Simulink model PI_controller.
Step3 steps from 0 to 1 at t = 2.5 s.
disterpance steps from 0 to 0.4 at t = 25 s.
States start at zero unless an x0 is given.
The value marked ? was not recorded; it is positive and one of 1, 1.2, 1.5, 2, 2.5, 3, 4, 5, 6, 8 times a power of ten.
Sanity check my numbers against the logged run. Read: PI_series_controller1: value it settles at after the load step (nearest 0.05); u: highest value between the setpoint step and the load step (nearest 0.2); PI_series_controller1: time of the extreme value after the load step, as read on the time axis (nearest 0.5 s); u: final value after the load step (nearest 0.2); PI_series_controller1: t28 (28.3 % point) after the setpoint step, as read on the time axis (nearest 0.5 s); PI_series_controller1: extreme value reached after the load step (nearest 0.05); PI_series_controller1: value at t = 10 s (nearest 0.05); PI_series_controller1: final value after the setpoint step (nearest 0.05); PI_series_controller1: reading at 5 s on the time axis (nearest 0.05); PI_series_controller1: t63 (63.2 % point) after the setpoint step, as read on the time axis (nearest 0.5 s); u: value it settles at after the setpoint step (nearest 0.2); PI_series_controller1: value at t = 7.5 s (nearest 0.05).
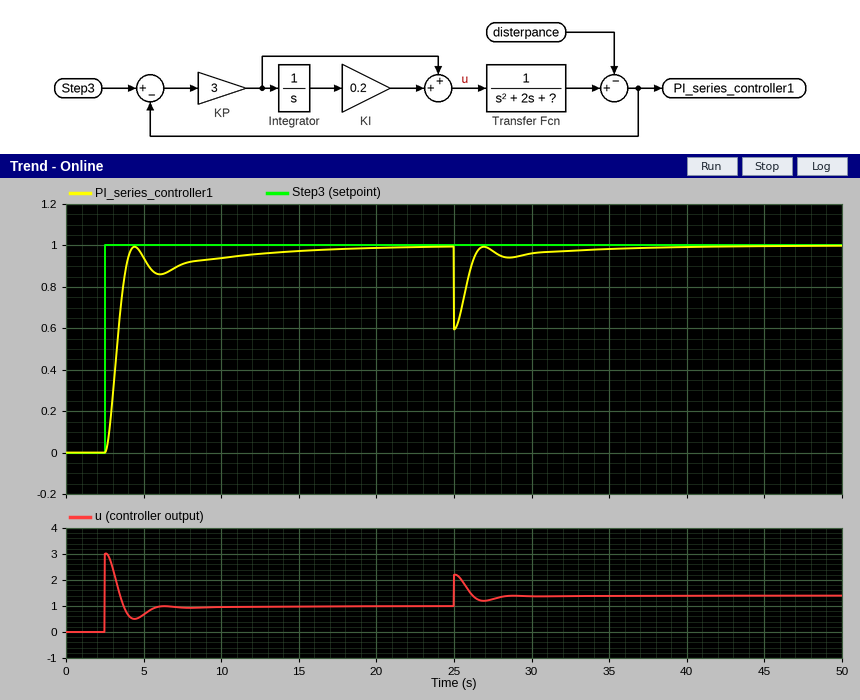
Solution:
1.00
3.0
25.0 s
1.4
3.0 s
0.60
0.95
1.00
0.95
3.5 s
1.0
0.90
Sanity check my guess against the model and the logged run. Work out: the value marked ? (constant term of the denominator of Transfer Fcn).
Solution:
1
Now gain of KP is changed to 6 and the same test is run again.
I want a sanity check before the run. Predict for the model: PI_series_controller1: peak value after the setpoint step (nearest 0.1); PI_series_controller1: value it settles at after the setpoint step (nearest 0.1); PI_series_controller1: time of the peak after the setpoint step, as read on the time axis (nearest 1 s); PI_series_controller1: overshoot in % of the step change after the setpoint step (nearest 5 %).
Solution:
1.2
1.0
4 s
20 %
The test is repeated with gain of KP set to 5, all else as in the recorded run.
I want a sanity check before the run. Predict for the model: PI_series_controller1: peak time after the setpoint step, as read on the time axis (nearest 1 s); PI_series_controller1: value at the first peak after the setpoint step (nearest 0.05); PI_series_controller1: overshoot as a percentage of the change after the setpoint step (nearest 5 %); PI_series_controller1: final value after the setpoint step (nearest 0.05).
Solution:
4 s
1.15
15 %
1.00
